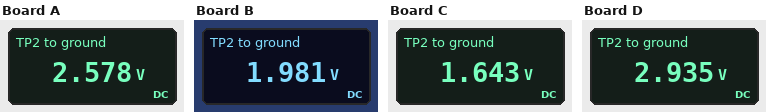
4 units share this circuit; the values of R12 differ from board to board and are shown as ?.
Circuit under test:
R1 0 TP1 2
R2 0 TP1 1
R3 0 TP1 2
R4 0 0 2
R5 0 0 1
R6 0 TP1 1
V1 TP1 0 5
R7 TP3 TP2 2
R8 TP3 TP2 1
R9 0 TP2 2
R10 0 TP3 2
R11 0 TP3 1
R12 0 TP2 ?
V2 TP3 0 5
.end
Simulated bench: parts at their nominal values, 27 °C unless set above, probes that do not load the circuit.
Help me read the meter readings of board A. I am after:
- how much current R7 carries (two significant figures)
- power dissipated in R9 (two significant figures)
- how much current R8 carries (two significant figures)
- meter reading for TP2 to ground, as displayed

1.2 A
3.3 W
2.4 A
2.578 V
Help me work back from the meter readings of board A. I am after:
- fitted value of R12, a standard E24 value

1.1 Ω
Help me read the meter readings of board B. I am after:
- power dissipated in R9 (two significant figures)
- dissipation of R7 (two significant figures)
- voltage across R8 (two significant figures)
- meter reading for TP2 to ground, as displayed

2.0 W
4.6 W
3.0 V
1.981 V
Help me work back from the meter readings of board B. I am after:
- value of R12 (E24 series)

0.56 Ω
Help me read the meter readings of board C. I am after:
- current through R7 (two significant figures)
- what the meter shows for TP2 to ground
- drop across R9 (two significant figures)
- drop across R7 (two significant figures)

1.7 A
1.643 V
1.6 V
3.4 V
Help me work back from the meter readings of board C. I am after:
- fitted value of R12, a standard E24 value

0.39 Ω
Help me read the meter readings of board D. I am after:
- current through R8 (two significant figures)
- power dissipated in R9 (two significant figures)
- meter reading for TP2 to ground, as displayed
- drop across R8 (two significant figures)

2.1 A
4.3 W
2.935 V
2.1 V
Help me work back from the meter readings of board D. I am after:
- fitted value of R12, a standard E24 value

1.8 Ω
